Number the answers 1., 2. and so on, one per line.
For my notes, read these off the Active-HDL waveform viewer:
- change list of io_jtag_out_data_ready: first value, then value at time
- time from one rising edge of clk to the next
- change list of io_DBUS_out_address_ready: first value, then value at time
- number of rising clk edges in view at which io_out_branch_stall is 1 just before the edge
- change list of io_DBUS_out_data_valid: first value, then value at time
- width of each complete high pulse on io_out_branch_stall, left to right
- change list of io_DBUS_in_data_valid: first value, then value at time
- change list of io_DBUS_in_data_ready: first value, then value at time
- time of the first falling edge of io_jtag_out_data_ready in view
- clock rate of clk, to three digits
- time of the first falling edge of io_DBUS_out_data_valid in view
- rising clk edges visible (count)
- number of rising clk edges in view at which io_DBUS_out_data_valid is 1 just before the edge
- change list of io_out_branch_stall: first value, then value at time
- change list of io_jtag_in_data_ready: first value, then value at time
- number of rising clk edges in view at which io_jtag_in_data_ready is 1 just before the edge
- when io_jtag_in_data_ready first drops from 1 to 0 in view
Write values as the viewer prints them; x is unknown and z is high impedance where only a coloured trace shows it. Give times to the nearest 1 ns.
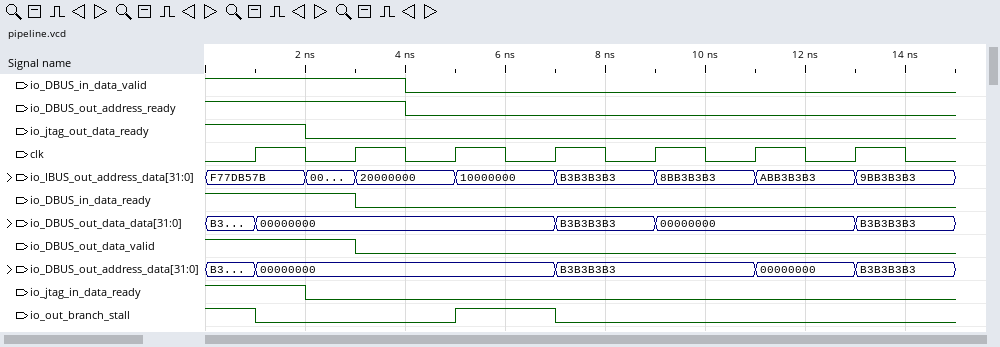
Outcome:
1. 1, 0 at 2 ns
2. 2 ns
3. 1, 0 at 4 ns
4. 2
5. 1, 0 at 3 ns
6. 2 ns
7. 1, 0 at 4 ns
8. 1, 0 at 3 ns
9. 2 ns
10. 500 MHz
11. 3 ns
12. 7
13. 2
14. 1, 0 at 1 ns, 1 at 5 ns, 0 at 7 ns
15. 1, 0 at 2 ns
16. 1
17. 2 ns
